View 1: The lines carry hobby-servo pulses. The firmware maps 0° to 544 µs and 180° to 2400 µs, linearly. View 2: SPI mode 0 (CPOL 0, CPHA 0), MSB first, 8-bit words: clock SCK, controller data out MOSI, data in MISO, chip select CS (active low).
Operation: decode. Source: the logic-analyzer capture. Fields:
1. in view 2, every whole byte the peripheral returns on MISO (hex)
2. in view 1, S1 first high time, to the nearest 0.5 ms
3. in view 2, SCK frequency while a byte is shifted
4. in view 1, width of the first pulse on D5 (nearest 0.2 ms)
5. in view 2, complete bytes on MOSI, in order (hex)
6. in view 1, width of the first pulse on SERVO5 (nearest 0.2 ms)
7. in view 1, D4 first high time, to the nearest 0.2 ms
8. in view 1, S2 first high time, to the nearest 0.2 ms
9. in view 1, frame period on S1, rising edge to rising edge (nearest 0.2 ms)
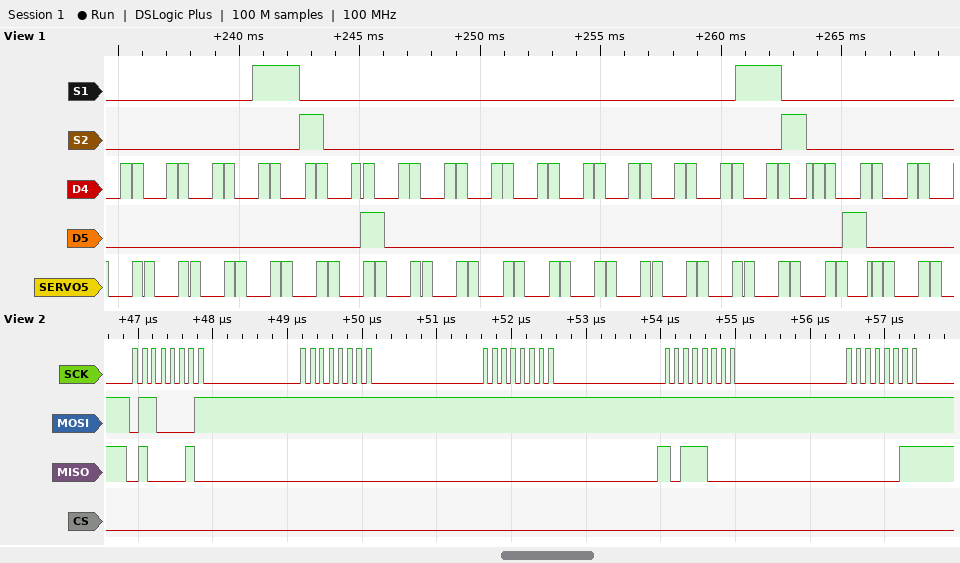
42 00 00 B8 03
2.0 ms
8 MHz
1.0 ms
61 FF FF FF FF
0.4 ms
0.4 ms
1.0 ms
20.0 ms
